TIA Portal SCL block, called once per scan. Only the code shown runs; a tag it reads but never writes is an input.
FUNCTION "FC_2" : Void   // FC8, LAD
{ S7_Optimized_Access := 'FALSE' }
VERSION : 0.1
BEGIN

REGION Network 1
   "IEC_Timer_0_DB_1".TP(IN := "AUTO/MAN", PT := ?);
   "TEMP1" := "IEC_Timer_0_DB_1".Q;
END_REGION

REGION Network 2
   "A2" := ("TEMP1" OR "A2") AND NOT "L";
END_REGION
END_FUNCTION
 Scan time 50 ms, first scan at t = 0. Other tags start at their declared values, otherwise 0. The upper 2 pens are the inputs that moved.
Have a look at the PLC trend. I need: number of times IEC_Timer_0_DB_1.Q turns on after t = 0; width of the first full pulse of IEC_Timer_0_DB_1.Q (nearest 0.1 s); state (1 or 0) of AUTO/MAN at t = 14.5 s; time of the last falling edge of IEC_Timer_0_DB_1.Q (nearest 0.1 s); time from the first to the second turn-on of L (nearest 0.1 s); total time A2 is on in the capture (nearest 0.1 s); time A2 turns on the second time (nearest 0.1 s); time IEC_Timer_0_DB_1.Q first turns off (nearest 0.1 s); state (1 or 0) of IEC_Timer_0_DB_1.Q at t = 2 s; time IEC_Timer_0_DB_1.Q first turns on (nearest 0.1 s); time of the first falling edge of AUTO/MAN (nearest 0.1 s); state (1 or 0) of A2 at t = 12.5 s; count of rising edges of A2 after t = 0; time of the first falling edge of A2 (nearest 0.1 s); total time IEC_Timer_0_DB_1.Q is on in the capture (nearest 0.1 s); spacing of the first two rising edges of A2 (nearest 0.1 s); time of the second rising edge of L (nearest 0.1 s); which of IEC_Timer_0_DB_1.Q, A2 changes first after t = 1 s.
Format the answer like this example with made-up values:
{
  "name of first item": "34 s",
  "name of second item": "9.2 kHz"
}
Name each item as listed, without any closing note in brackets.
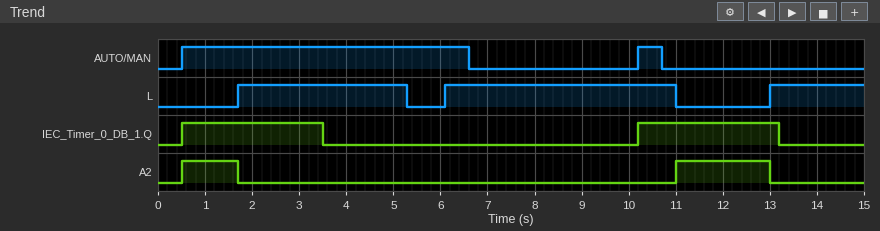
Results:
{
  "number of times IEC_Timer_0_DB_1.Q turns on after t = 0": "2",
  "width of the first full pulse of IEC_Timer_0_DB_1.Q": "3.0 s",
  "state (1 or 0) of AUTO/MAN at t = 14.5 s": "0",
  "time of the last falling edge of IEC_Timer_0_DB_1.Q": "13.2 s",
  "time from the first to the second turn-on of L": "4.4 s",
  "total time A2 is on in the capture": "3.2 s",
  "time A2 turns on the second time": "11.0 s",
  "time IEC_Timer_0_DB_1.Q first turns off": "3.5 s",
  "state (1 or 0) of IEC_Timer_0_DB_1.Q at t = 2 s": "1",
  "time IEC_Timer_0_DB_1.Q first turns on": "0.5 s",
  "time of the first falling edge of AUTO/MAN": "6.6 s",
  "state (1 or 0) of A2 at t = 12.5 s": "1",
  "count of rising edges of A2 after t = 0": "2",
  "time of the first falling edge of A2": "1.7 s",
  "total time IEC_Timer_0_DB_1.Q is on in the capture": "6.0 s",
  "spacing of the first two rising edges of A2": "10.5 s",
  "time of the second rising edge of L": "6.1 s",
  "which of IEC_Timer_0_DB_1.Q, A2 changes first after t = 1 s": "A2"
}
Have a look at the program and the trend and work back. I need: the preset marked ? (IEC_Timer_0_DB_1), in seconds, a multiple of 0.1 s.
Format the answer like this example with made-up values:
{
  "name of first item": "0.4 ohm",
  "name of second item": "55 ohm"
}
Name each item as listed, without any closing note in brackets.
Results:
{
  "the preset marked ? (IEC_Timer_0_DB_1), in seconds, a multiple of 0.1 s": "3.0 s"
}
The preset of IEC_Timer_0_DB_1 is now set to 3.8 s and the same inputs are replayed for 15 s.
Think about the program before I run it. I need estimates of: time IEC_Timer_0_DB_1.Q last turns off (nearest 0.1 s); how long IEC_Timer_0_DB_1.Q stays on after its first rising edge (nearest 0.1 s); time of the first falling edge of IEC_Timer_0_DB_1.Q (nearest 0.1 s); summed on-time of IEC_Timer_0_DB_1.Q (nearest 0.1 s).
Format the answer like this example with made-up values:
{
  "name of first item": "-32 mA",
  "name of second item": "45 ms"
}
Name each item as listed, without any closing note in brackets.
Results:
{
  "time IEC_Timer_0_DB_1.Q last turns off": "14.0 s",
  "how long IEC_Timer_0_DB_1.Q stays on after its first rising edge": "3.8 s",
  "time of the first falling edge of IEC_Timer_0_DB_1.Q": "4.3 s",
  "summed on-time of IEC_Timer_0_DB_1.Q": "7.6 s"
}
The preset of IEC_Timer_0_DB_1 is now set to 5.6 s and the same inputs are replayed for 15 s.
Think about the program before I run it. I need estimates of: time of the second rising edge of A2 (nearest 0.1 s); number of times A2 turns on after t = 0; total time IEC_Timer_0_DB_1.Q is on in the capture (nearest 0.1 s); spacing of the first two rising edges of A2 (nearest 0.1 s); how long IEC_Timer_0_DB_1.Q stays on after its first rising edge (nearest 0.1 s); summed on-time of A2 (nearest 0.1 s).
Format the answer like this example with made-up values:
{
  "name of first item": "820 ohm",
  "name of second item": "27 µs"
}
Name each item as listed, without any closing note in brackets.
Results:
{
  "time of the second rising edge of A2": "5.3 s",
  "number of times A2 turns on after t = 0": "3",
  "total time IEC_Timer_0_DB_1.Q is on in the capture": "10.4 s",
  "spacing of the first two rising edges of A2": "4.8 s",
  "how long IEC_Timer_0_DB_1.Q stays on after its first rising edge": "5.6 s",
  "summed on-time of A2": "4.0 s"
}
